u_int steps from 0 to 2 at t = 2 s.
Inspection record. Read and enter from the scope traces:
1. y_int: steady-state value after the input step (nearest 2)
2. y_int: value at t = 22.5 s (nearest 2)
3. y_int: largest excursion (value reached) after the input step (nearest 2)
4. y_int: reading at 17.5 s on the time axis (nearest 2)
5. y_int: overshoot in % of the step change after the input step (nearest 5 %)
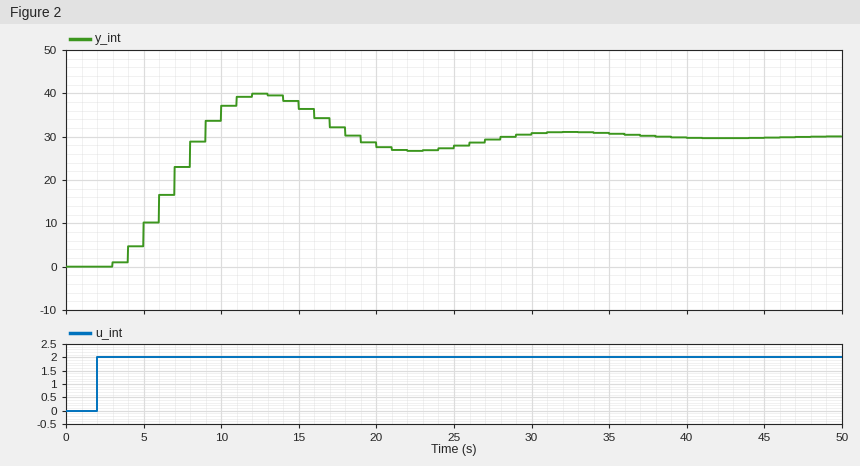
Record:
30
26
40
32
35 %
